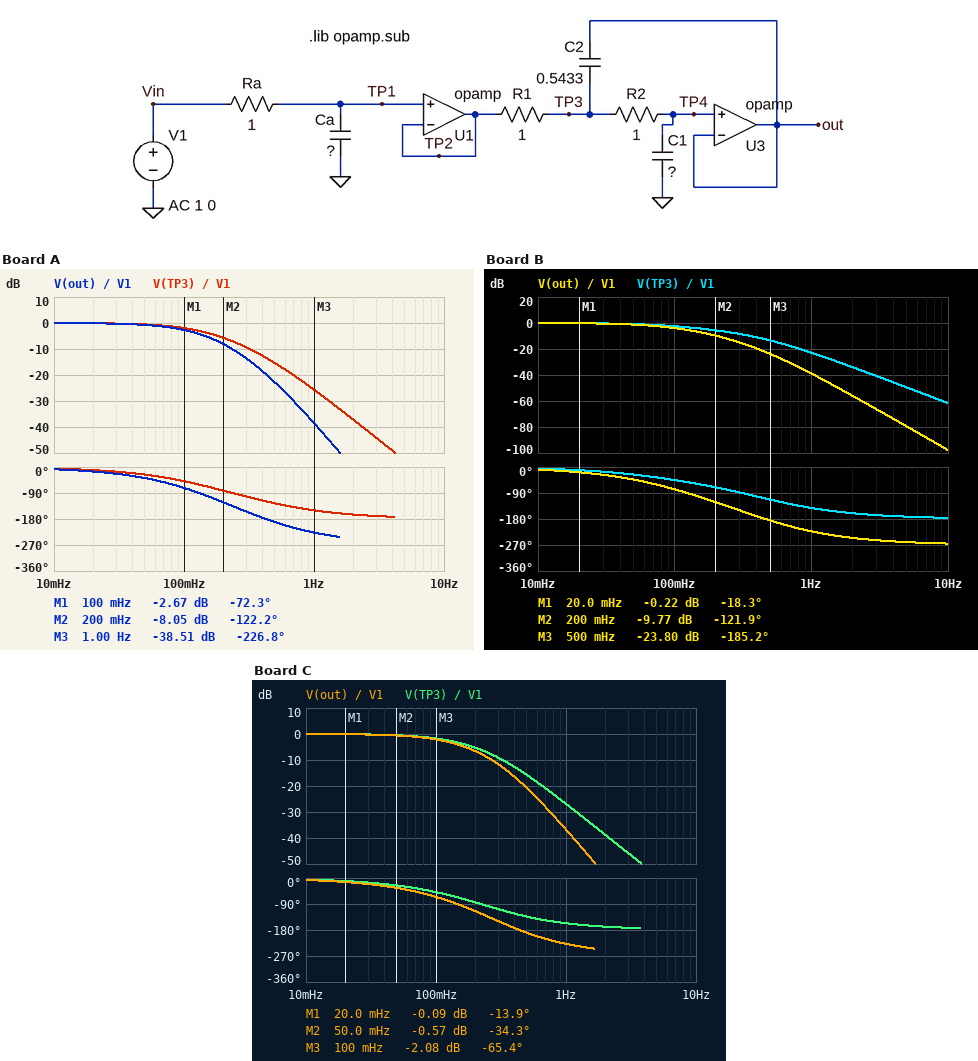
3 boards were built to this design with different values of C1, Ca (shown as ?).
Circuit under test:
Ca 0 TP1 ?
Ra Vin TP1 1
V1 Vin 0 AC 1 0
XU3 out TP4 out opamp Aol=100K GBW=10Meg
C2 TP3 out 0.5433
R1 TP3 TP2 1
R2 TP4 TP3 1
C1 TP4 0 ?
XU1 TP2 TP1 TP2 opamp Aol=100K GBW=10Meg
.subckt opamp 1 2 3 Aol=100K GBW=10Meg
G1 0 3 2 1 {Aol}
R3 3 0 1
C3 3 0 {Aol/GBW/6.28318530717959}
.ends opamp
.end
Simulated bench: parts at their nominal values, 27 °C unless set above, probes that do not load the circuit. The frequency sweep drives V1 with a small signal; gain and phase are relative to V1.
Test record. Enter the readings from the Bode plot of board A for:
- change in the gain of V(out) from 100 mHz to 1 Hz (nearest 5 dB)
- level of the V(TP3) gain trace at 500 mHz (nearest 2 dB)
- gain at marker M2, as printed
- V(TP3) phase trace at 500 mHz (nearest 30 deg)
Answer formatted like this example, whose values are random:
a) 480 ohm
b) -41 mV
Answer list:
a) -35 dB
b) -16 dB
c) -8.05 dB
d) -120 deg
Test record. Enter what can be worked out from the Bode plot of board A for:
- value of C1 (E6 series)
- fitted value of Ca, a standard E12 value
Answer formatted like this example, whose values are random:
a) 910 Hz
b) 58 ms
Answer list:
a) 680 mF
b) 820 mF
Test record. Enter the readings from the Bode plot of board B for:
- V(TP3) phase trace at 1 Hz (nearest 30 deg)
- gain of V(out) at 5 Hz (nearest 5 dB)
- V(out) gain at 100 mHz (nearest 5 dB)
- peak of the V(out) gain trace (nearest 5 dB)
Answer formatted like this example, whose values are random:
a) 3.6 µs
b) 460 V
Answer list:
a) -150 deg
b) -80 dB
c) -5 dB
d) 0 dB
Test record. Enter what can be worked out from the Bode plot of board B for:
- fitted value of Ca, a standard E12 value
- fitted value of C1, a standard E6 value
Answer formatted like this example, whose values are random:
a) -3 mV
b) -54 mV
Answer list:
a) 560 mF
b) 1 F
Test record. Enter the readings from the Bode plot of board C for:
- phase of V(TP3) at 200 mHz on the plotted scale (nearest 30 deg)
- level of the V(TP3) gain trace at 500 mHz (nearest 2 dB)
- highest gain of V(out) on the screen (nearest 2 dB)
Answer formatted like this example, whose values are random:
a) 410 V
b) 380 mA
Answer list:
a) -90 deg
b) -16 dB
c) 0 dB
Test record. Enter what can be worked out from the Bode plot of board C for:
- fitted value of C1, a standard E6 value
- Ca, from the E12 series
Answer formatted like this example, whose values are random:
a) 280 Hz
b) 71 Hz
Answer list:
a) 470 mF
b) 1 F
